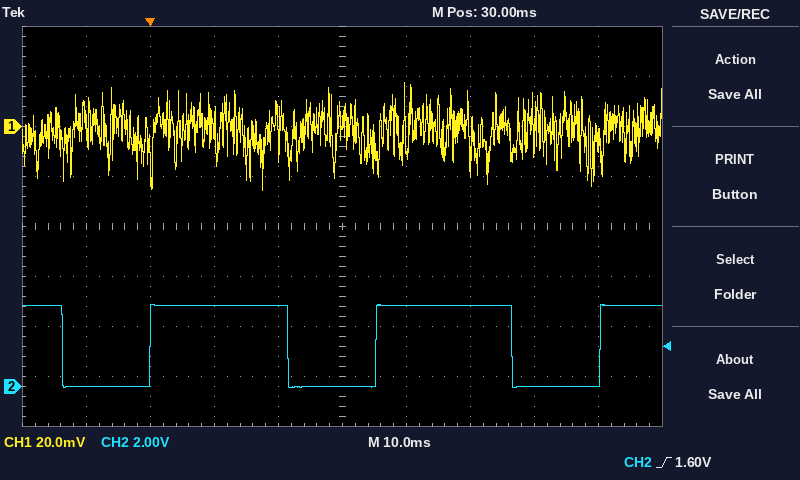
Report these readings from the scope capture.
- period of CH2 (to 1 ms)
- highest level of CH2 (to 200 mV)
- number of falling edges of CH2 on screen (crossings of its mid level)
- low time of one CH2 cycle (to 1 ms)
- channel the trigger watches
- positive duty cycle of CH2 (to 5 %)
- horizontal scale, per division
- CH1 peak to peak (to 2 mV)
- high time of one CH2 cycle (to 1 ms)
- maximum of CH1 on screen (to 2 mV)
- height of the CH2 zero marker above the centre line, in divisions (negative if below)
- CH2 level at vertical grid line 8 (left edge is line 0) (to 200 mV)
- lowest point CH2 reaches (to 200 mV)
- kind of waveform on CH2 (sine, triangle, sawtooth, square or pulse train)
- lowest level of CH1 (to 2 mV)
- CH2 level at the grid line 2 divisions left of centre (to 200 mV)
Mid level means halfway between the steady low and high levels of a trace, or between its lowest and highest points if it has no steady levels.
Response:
35 ms
3.2 V
3
14 ms
CH2
60 %
10 ms
44 mV
21 ms
18 mV
-3.2 div
0.0 V
0.0 V
pulse train
-26 mV
3.2 V
